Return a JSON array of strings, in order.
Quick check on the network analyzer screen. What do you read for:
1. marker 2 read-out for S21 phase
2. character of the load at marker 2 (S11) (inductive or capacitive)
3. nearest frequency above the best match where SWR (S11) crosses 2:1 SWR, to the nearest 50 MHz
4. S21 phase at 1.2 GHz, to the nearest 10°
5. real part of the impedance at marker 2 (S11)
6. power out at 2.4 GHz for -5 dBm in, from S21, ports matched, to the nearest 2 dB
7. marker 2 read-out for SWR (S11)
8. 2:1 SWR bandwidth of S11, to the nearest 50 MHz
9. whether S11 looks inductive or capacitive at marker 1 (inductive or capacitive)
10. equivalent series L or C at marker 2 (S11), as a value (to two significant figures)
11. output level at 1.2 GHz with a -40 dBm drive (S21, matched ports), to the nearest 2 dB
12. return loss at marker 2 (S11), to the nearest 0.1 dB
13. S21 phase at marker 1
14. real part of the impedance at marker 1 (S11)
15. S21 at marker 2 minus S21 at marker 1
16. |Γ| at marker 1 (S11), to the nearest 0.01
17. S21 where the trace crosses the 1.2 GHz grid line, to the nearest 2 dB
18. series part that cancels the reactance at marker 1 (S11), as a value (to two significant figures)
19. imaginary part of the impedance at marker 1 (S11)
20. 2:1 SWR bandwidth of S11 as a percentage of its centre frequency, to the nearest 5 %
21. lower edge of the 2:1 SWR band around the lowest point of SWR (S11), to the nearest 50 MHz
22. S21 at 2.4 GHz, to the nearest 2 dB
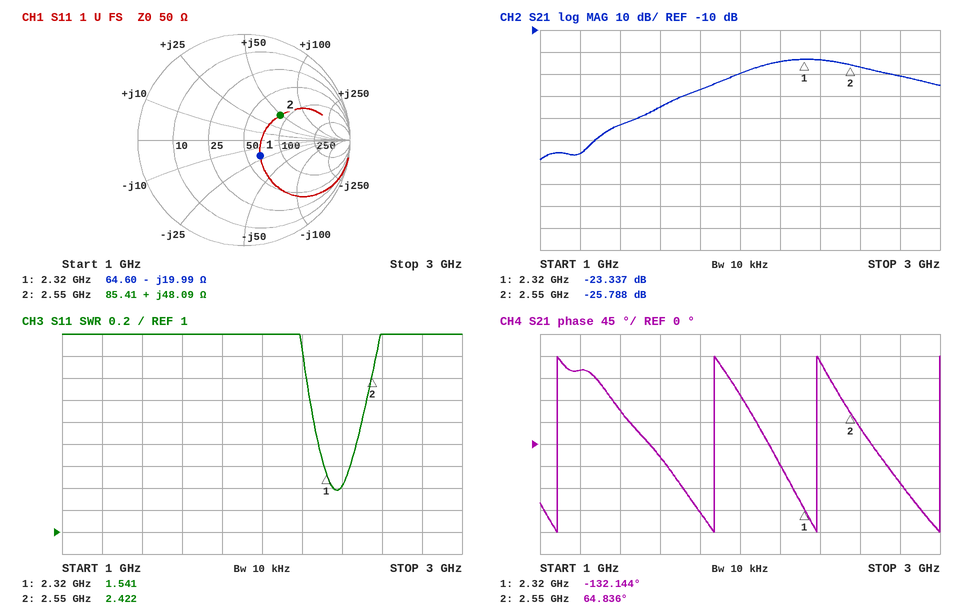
["64.836°", "inductive", "2.50 GHz", "150°", "85.41 Ω", "-28 dBm", "2.422", "250 MHz", "capacitive", "3.0 nH", "-106 dBm", "7.6 dB", "-132.144°", "64.60 Ω", "-2.451 dB", "0.21", "-66 dB", "1.4 nH", "-19.99 Ω", "10 %", "2.25 GHz", "-24 dB"]
